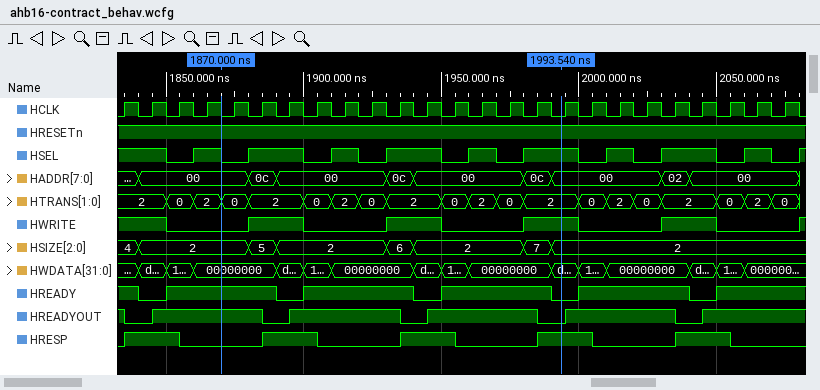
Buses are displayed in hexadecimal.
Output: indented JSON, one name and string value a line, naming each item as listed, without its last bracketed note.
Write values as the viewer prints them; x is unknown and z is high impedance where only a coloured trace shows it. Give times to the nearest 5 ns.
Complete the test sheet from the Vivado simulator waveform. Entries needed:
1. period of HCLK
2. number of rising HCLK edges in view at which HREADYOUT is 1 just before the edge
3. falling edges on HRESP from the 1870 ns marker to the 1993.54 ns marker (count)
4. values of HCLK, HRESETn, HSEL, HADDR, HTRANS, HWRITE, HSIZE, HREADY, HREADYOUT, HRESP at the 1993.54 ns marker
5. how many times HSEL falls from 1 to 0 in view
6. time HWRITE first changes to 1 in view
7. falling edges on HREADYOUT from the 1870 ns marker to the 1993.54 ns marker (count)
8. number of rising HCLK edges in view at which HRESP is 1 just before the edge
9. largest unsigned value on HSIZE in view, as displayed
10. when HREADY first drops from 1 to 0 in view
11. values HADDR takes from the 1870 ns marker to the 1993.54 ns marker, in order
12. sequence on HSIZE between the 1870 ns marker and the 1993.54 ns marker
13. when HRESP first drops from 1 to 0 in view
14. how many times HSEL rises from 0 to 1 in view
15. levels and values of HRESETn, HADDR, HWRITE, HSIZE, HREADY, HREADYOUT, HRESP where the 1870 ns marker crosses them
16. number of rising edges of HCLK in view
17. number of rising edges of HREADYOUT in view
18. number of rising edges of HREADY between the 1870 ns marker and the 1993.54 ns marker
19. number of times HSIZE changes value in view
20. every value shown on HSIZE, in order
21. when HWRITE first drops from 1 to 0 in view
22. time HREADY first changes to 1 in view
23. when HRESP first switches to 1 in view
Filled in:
{
  "period of HCLK": "10 ns",
  "number of rising HCLK edges in view at which HREADYOUT is 1 just before the edge": "20",
  "falling edges on HRESP from the 1870 ns marker to the 1993.54 ns marker": "2",
  "values of HCLK, HRESETn, HSEL, HADDR, HTRANS, HWRITE, HSIZE, HREADY, HREADYOUT, HRESP at the 1993.54 ns marker": "HCLK=0, HRESETn=1, HSEL=1, HADDR=00, HTRANS=2, HWRITE=1, HSIZE=2, HREADY=0, HREADYOUT=0, HRESP=1",
  "how many times HSEL falls from 1 to 0 in view": "10",
  "time HWRITE first changes to 1 in view": "1880 ns",
  "falling edges on HREADYOUT from the 1870 ns marker to the 1993.54 ns marker": "3",
  "number of rising HCLK edges in view at which HRESP is 1 just before the edge": "10",
  "largest unsigned value on HSIZE in view, as displayed": "7",
  "when HREADY first drops from 1 to 0 in view": "1840 ns",
  "values HADDR takes from the 1870 ns marker to the 1993.54 ns marker, in order": "00, 0c, 00, 0c, 00, 0c, 00",
  "sequence on HSIZE between the 1870 ns marker and the 1993.54 ns marker": "2, 5, 2, 6, 2, 7, 2",
  "when HRESP first drops from 1 to 0 in view": "1855 ns",
  "how many times HSEL rises from 0 to 1 in view": "10",
  "levels and values of HRESETn, HADDR, HWRITE, HSIZE, HREADY, HREADYOUT, HRESP where the 1870 ns marker crosses them": "HRESETn=1, HADDR=00, HWRITE=0, HSIZE=2, HREADY=1, HREADYOUT=1, HRESP=0",
  "number of rising edges of HCLK in view": "25",
  "number of rising edges of HREADYOUT in view": "5",
  "number of rising edges of HREADY between the 1870 ns marker and the 1993.54 ns marker": "2",
  "number of times HSIZE changes value in view": "7",
  "every value shown on HSIZE, in order": "4, 2, 5, 2, 6, 2, 7, 2",
  "when HWRITE first drops from 1 to 0 in view": "1850 ns",
  "time HREADY first changes to 1 in view": "1850 ns",
  "when HRESP first switches to 1 in view": "1835 ns"
}
